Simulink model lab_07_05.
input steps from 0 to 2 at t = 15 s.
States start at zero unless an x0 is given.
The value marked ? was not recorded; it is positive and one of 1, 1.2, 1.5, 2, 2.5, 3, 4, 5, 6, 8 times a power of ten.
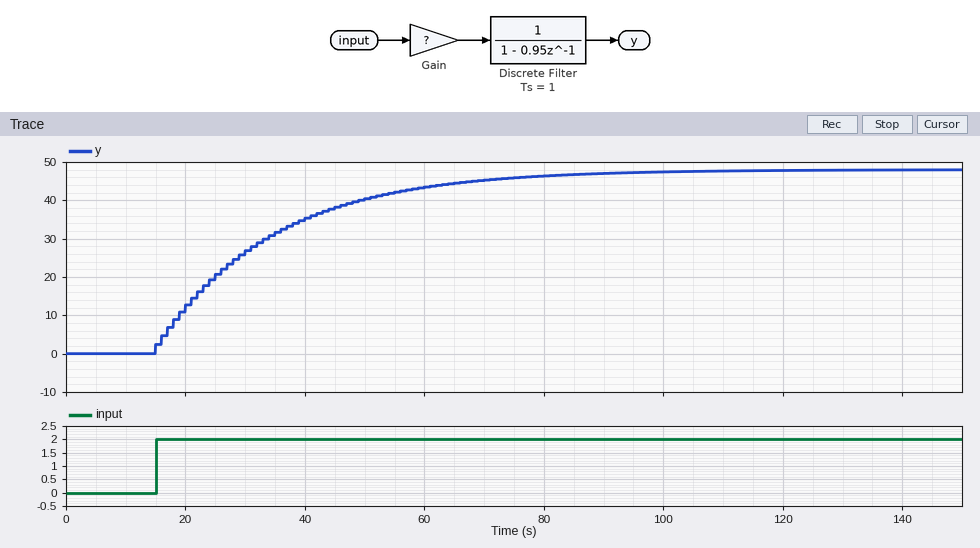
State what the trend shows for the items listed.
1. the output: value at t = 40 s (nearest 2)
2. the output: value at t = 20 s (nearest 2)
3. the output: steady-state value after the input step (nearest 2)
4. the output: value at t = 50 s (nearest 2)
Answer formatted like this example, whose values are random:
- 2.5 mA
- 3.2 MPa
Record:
- 36
- 12
- 48
- 40
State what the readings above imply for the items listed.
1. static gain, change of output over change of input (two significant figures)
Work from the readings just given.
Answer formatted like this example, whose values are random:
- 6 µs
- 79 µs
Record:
- 24
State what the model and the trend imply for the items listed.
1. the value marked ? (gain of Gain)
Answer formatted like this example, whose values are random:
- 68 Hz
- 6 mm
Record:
- 1.2
